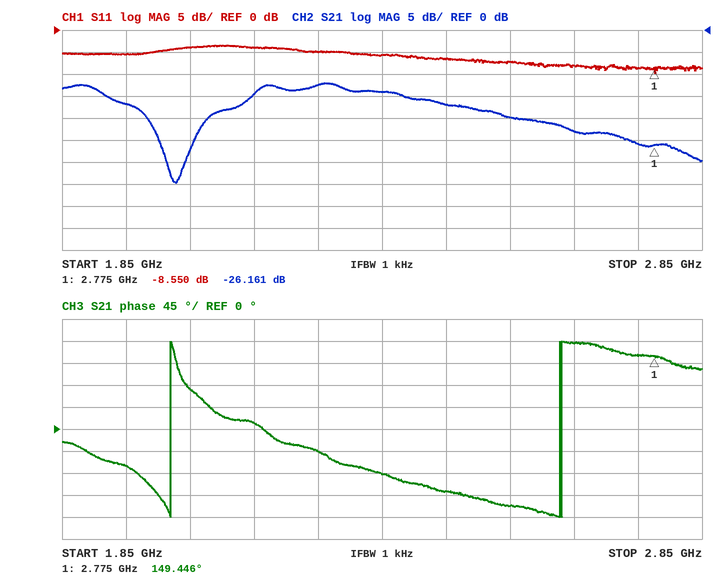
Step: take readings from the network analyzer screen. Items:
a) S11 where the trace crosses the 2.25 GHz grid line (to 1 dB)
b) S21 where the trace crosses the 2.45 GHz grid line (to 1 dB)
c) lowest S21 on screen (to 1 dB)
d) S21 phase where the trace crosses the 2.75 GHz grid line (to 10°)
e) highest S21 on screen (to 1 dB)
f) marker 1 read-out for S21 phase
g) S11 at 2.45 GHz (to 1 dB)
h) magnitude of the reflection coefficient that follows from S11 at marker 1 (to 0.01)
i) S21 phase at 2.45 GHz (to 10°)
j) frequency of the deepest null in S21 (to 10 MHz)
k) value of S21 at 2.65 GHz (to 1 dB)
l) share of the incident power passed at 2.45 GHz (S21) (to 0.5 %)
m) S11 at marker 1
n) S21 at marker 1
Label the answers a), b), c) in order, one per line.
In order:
a) -5 dB
b) -17 dB
c) -35 dB
d) 150°
e) -12 dB
f) 149.446°
g) -7 dB
h) 0.37
i) -130°
j) 2.03 GHz
k) -23 dB
l) 2.0 %
m) -8.550 dB
n) -26.161 dB
